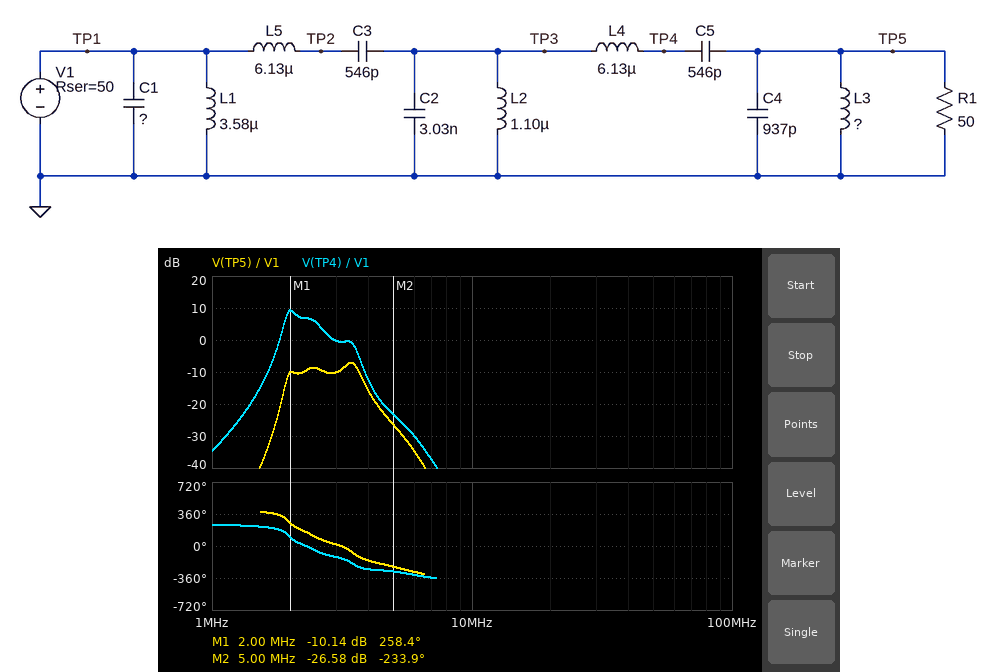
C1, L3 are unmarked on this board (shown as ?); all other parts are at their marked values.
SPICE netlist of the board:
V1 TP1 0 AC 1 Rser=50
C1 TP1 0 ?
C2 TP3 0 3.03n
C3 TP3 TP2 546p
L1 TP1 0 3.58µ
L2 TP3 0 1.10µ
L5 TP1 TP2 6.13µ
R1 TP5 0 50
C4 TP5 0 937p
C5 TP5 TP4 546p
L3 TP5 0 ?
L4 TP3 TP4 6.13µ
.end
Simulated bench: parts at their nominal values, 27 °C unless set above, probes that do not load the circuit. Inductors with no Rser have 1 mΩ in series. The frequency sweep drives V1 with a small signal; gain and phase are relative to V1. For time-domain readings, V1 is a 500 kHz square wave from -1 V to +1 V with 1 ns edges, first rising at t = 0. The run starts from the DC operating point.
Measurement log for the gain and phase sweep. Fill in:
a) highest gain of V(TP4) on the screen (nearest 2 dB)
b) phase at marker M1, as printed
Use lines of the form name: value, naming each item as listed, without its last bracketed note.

highest gain of V(TP4) on the screen: 10 dB
phase at marker M1, as printed: 258.4 deg
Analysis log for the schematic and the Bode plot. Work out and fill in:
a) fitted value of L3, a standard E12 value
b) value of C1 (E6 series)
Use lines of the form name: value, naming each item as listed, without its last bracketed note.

fitted value of L3, a standard E12 value: 1 µH
value of C1: 470 pF
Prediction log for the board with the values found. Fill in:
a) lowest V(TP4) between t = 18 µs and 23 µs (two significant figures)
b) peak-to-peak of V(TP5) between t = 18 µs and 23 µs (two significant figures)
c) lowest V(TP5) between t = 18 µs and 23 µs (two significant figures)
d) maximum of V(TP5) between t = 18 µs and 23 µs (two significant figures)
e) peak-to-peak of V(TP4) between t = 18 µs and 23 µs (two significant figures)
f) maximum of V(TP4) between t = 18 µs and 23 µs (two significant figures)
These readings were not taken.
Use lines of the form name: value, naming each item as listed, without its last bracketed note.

lowest V(TP4) between t = 18 µs and 23 µs: -630 mV
peak-to-peak of V(TP5) between t = 18 µs and 23 µs: 340 mV
lowest V(TP5) between t = 18 µs and 23 µs: -170 mV
maximum of V(TP5) between t = 18 µs and 23 µs: 170 mV
peak-to-peak of V(TP4) between t = 18 µs and 23 µs: 1.3 V
maximum of V(TP4) between t = 18 µs and 23 µs: 630 mV
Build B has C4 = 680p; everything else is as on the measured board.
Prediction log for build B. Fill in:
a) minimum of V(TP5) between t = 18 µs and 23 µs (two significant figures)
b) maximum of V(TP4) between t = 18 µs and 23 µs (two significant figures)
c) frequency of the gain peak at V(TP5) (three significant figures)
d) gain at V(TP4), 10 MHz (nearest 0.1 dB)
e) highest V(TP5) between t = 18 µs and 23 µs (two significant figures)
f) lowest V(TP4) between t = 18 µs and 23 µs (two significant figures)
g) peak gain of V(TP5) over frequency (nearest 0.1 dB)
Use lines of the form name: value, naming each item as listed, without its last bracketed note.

minimum of V(TP5) between t = 18 µs and 23 µs: -160 mV
maximum of V(TP4) between t = 18 µs and 23 µs: 670 mV
frequency of the gain peak at V(TP5): 3.44 MHz
gain at V(TP4), 10 MHz: -54.6 dB
highest V(TP5) between t = 18 µs and 23 µs: 160 mV
lowest V(TP4) between t = 18 µs and 23 µs: -670 mV
peak gain of V(TP5) over frequency: -7.5 dB
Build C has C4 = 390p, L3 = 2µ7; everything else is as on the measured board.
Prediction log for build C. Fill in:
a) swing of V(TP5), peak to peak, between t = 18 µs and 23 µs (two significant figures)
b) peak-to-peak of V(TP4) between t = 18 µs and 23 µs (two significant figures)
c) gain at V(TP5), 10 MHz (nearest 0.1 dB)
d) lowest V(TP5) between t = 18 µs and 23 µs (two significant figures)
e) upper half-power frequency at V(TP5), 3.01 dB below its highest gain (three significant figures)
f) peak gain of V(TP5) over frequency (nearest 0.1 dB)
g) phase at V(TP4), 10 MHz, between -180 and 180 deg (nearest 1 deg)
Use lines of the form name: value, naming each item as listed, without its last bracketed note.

swing of V(TP5), peak to peak, between t = 18 µs and 23 µs: 410 mV
peak-to-peak of V(TP4) between t = 18 µs and 23 µs: 900 mV
gain at V(TP5), 10 MHz: -58.3 dB
lowest V(TP5) between t = 18 µs and 23 µs: -210 mV
upper half-power frequency at V(TP5), 3.01 dB below its highest gain: 3.71 MHz
peak gain of V(TP5) over frequency: -6.1 dB
phase at V(TP4), 10 MHz, between -180 and 180 deg: -17 deg
